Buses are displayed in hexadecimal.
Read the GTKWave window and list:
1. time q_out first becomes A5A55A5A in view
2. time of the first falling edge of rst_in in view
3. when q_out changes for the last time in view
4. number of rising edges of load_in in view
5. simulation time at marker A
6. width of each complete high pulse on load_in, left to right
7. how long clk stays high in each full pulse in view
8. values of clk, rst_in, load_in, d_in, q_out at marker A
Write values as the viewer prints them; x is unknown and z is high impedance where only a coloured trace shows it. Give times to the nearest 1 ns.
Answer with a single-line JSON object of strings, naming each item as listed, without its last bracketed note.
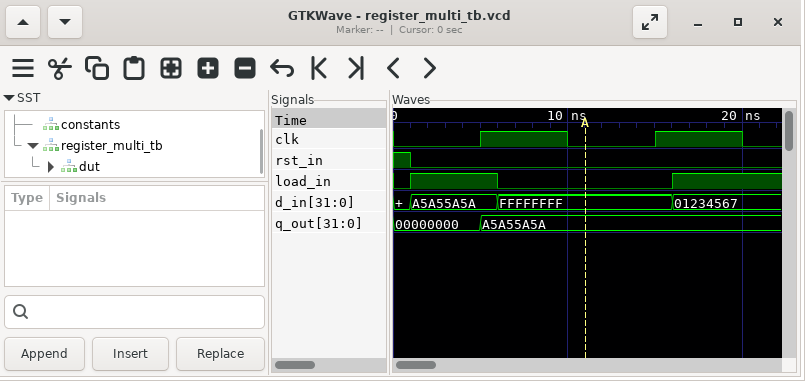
{"time q_out first becomes A5A55A5A in view": "5 ns", "time of the first falling edge of rst_in in view": "1 ns", "when q_out changes for the last time in view": "5 ns", "number of rising edges of load_in in view": "2", "simulation time at marker A": "11 ns", "width of each complete high pulse on load_in, left to right": "5 ns", "how long clk stays high in each full pulse in view": "5 ns, 5 ns", "values of clk, rst_in, load_in, d_in, q_out at marker A": "clk=0, rst_in=0, load_in=0, d_in=FFFFFFFF, q_out=A5A55A5A"}
